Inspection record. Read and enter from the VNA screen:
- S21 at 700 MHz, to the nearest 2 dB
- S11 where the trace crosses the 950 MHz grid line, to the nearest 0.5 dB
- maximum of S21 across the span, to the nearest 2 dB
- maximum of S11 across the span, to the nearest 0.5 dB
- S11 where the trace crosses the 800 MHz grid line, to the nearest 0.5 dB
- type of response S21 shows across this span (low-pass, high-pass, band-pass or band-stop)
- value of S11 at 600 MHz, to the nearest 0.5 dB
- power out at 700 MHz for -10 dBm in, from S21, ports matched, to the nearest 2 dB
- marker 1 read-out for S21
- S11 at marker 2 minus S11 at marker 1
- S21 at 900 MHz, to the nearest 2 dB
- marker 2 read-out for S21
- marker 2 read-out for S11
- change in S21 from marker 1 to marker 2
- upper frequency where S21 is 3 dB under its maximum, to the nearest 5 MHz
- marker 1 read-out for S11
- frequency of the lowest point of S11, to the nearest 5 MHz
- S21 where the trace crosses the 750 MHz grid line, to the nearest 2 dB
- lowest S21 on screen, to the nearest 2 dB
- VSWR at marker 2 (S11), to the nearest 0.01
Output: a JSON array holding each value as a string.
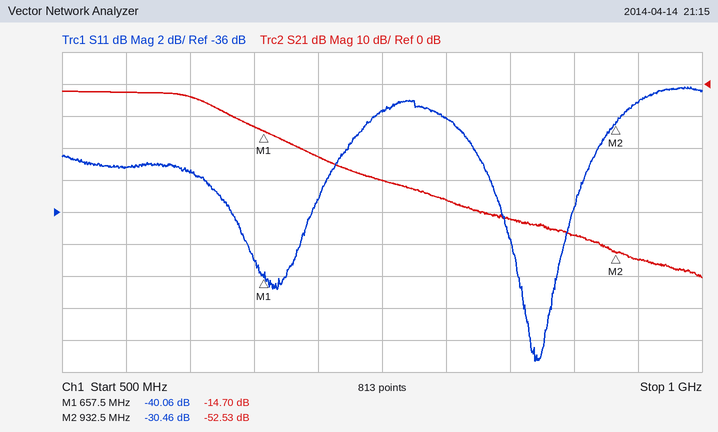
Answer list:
["-22 dB", "-29.0 dB", "-2 dB", "-28.0 dB", "-30.0 dB", "low-pass", "-33.5 dB", "-32 dBm", "-14.70 dB", "9.60 dB", "-48 dB", "-52.53 dB", "-30.46 dB", "-37.83 dB", "610 MHz", "-40.06 dB", "870 MHz", "-30 dB", "-60 dB", "1.06"]
